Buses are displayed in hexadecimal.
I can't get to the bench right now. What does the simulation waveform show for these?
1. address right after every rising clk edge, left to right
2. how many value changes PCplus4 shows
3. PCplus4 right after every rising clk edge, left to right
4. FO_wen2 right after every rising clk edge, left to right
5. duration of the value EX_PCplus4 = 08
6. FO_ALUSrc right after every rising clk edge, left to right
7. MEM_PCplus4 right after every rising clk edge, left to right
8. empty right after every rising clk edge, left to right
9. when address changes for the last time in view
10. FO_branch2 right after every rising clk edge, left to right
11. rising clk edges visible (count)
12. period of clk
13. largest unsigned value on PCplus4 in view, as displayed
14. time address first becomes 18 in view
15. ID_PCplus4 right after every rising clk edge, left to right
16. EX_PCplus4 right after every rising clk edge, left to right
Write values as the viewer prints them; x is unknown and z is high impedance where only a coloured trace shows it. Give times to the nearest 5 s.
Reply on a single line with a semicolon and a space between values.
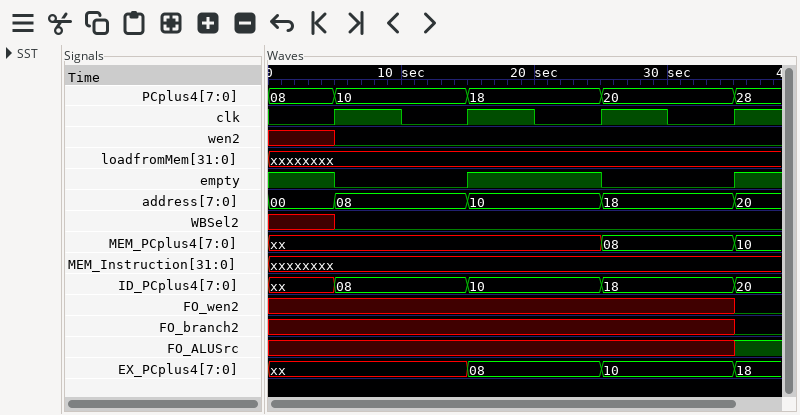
08, 10, 18, 20; 4; 10, 18, 20, 28; x x x 0; 10 s; x x x 1; xx, xx, 08, 10; 0 1 0 1; 35 s; x x x 0; 4; 10 s; 28; 25 s; 08, 10, 18, 20; xx, 08, 10, 18
